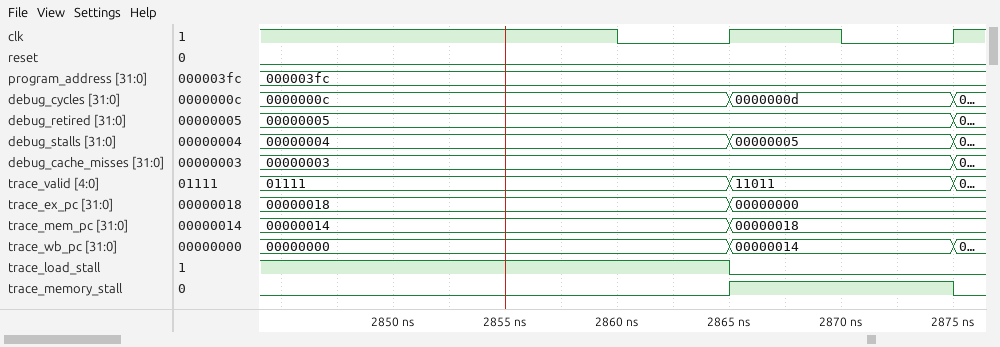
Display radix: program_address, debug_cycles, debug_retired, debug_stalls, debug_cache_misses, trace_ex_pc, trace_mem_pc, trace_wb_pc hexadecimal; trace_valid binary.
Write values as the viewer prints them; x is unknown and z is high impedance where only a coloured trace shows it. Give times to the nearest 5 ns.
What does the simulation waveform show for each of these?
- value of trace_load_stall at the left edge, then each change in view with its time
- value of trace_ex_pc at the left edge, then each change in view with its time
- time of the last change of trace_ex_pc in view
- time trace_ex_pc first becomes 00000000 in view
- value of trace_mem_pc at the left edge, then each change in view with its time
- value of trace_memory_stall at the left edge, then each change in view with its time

1, 0 at 2865 ns
00000018, 00000000 at 2865 ns
2865 ns
2865 ns
00000014, 00000018 at 2865 ns
0, 1 at 2865 ns, 0 at 2875 ns
